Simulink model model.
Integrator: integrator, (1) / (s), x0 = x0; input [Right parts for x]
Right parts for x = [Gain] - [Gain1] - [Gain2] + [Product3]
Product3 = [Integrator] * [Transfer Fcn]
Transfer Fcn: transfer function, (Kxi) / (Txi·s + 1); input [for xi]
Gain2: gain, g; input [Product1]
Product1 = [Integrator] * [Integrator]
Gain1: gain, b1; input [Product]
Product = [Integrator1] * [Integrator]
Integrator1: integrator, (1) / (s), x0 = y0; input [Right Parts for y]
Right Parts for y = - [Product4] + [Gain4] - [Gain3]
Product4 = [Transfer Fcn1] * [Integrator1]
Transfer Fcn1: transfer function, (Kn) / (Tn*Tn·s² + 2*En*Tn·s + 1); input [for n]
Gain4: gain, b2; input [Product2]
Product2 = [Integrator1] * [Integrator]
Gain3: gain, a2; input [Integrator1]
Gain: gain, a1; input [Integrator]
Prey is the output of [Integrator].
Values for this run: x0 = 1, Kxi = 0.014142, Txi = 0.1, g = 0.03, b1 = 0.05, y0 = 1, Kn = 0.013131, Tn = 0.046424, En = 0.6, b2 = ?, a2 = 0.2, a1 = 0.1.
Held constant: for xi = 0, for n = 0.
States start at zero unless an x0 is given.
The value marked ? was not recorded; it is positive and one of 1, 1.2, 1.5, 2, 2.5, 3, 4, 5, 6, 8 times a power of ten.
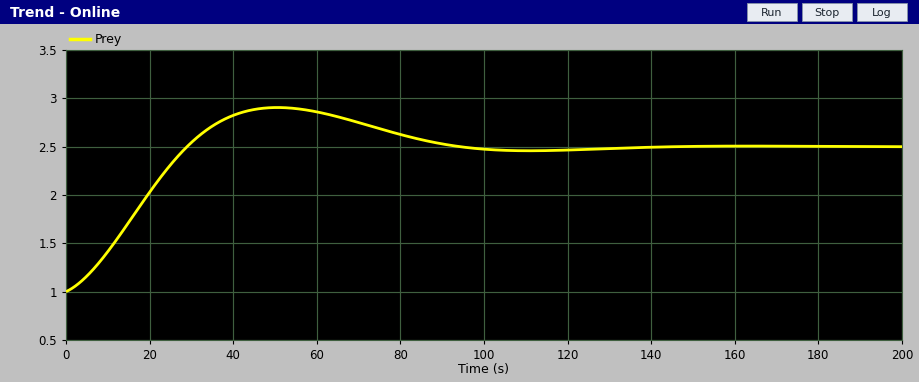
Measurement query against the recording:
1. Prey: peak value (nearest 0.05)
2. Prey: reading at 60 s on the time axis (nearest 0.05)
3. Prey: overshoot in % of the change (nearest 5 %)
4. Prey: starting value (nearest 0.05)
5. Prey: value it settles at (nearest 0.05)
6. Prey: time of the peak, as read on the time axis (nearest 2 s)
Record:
2.90
2.85
25 %
1.00
2.50
50 s
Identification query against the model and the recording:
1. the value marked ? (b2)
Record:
0.08
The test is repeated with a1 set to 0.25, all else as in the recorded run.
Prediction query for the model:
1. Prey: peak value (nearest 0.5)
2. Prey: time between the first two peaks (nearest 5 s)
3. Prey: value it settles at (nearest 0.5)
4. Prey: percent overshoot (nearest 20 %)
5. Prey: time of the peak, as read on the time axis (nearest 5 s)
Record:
5.0
35 s
2.5
160 %
15 s
